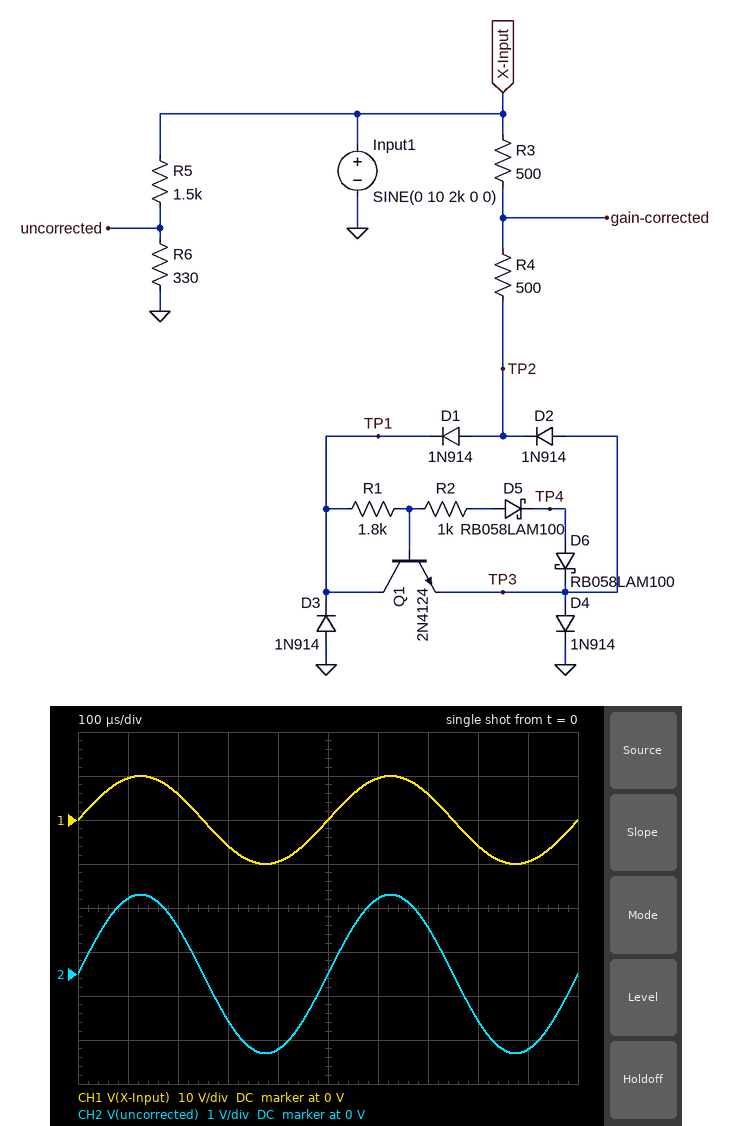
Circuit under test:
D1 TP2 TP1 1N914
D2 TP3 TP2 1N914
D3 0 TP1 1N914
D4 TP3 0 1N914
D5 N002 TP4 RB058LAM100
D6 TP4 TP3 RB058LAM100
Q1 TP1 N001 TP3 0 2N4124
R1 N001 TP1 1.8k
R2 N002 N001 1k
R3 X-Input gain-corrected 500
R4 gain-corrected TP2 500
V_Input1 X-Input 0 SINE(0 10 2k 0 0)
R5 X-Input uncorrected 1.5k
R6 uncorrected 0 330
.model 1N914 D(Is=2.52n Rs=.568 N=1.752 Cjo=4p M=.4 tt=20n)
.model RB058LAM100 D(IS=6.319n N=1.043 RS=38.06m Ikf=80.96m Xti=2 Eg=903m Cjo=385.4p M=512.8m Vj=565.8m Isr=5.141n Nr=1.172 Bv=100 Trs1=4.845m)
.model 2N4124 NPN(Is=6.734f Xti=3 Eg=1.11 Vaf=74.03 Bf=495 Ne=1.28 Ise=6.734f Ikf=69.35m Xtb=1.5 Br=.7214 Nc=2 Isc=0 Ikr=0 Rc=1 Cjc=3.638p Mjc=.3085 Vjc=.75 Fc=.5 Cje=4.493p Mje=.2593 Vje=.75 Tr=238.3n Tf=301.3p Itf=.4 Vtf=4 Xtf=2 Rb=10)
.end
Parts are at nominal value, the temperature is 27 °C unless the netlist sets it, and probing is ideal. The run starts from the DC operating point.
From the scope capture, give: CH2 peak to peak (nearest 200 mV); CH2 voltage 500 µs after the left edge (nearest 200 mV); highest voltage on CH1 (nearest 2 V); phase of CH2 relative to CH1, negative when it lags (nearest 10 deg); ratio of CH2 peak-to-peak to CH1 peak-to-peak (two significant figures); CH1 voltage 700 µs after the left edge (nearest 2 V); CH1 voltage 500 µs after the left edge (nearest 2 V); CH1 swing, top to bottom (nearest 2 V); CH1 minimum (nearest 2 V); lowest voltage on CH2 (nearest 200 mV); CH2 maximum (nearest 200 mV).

3.6 V
0 V
10 V
0 deg
0.18
6 V
0 V
20 V
-10 V
-1.8 V
1.8 V
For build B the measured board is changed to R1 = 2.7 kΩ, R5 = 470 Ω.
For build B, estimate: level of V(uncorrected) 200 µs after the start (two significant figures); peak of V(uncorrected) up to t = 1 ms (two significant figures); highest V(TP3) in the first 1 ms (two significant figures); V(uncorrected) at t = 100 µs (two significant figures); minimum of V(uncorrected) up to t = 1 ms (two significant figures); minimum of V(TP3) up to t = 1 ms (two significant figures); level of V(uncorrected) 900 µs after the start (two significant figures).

2.4 V
4.1 V
680 mV
3.9 V
-4.1 V
-2.0 V
-3.9 V
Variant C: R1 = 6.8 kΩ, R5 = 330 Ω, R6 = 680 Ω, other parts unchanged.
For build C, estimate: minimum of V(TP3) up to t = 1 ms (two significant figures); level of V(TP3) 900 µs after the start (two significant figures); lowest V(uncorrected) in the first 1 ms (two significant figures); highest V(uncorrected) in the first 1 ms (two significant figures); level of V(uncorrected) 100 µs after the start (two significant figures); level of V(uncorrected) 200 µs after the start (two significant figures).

-2.8 V
-2.7 V
-6.7 V
6.7 V
6.4 V
4.0 V
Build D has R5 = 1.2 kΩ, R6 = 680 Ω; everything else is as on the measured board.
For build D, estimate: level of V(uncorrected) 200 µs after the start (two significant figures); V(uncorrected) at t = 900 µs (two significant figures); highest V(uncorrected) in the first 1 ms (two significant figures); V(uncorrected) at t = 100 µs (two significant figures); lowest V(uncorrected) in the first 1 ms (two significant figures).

2.1 V
-3.4 V
3.6 V
3.4 V
-3.6 V
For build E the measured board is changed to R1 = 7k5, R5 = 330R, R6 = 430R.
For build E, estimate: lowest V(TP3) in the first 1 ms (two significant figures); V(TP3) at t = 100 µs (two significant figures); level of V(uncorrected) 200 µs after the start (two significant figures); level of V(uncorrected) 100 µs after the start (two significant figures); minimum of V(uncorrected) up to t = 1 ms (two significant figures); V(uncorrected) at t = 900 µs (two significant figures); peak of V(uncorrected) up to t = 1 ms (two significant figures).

-2.9 V
670 mV
3.3 V
5.4 V
-5.7 V
-5.4 V
5.7 V
